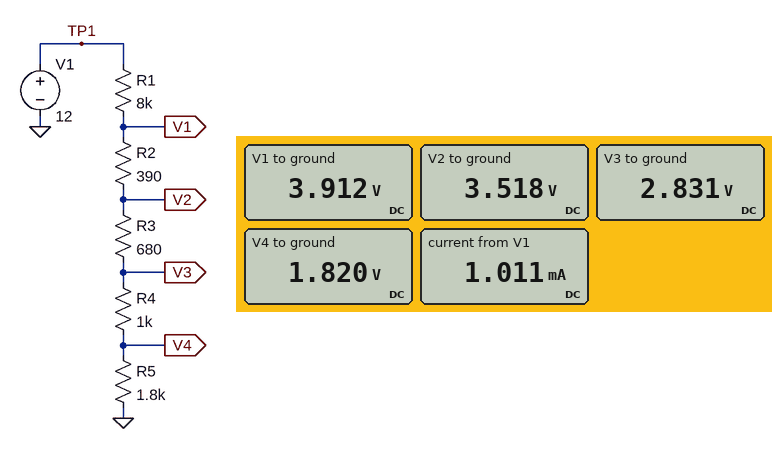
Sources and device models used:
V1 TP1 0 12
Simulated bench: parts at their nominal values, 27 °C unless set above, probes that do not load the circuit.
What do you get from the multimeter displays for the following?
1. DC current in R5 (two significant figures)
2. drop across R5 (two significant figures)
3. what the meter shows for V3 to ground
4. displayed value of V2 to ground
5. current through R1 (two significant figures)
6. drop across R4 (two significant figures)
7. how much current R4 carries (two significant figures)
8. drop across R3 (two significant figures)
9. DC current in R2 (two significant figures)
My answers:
1.0 mA
1.8 V
2.831 V
3.518 V
1.0 mA
1.0 V
1.0 mA
690 mV
1.0 mA
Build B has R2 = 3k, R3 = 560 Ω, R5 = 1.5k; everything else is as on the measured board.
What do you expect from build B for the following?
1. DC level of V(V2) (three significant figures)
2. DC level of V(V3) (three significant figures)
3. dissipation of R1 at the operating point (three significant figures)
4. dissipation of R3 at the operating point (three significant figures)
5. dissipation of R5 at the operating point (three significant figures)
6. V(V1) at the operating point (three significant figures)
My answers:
2.61 V
2.13 V
5.83 mW
408 µW
1.09 mW
5.17 V
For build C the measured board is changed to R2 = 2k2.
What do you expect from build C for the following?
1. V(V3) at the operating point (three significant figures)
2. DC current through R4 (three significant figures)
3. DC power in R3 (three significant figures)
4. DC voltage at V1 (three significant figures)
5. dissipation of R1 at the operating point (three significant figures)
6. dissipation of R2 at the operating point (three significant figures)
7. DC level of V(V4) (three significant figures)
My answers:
2.46 V
877 µA
523 µW
4.98 V
6.16 mW
1.69 mW
1.58 V
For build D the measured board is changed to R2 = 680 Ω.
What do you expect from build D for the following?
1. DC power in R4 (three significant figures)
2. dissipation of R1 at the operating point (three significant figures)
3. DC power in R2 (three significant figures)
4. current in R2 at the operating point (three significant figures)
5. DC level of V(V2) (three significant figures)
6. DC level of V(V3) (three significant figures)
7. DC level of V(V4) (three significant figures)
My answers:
974 µW
7.79 mW
662 µW
987 µA
3.43 V
2.76 V
1.78 V
